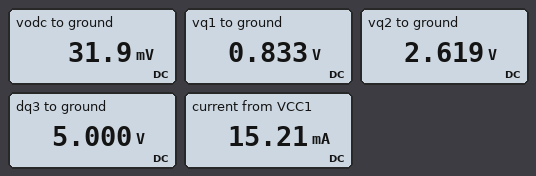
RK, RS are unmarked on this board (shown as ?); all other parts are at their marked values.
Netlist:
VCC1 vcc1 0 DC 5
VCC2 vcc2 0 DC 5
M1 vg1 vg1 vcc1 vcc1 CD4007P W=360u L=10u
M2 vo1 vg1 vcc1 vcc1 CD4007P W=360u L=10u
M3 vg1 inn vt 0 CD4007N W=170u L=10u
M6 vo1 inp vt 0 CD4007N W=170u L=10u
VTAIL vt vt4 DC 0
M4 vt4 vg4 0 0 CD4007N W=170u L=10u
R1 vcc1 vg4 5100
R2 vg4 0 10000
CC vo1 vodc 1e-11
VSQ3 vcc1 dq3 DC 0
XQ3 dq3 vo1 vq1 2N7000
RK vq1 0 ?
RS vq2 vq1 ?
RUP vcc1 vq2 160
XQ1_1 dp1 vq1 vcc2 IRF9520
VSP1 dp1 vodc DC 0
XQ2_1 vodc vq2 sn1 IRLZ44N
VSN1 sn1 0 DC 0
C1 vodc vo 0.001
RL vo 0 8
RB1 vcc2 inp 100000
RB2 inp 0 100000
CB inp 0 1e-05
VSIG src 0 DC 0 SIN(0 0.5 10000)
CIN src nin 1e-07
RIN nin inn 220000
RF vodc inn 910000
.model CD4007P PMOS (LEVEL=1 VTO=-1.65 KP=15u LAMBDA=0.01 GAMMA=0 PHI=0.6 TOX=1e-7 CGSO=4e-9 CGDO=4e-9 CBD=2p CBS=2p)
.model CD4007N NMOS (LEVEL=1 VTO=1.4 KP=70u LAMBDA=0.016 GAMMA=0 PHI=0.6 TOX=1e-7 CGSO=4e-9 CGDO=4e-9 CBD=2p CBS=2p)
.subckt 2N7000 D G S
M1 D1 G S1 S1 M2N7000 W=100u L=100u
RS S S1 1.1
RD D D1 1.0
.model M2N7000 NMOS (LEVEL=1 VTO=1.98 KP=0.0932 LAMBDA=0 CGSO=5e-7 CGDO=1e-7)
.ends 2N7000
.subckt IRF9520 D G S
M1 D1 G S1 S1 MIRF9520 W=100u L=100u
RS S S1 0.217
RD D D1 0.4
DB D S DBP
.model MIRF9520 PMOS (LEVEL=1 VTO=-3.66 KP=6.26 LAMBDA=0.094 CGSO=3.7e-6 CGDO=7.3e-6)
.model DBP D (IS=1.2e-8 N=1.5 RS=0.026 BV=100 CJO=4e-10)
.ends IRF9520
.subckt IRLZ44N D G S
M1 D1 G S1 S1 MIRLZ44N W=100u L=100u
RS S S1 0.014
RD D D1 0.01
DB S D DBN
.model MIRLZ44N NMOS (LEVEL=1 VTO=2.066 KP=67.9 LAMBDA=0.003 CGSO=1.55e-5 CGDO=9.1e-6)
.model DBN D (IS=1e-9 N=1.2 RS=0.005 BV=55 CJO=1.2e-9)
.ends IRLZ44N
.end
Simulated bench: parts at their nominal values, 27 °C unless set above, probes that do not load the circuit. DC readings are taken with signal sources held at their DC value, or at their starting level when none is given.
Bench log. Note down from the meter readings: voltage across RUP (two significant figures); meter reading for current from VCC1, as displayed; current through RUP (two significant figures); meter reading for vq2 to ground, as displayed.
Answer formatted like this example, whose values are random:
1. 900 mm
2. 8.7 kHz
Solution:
1. 2.4 V
2. 15.21 mA
3. 15 mA
4. 2.619 V
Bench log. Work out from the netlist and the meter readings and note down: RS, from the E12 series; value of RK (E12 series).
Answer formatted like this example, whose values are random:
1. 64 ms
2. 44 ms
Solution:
1. 120 Ω
2. 56 Ω
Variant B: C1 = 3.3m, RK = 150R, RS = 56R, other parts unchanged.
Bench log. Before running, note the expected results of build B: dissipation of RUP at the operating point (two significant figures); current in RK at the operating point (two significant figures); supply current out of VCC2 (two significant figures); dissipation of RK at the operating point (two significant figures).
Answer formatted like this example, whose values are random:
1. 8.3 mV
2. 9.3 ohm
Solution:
1. 30 mW
2. 14 mA
3. 25 µA
4. 28 mW
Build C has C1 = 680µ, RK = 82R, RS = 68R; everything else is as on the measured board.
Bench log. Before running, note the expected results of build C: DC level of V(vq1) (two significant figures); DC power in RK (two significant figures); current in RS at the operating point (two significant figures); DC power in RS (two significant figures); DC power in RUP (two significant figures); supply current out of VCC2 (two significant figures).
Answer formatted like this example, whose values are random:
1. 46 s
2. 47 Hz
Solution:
1. 1.3 V
2. 21 mW
3. 16 mA
4. 18 mW
5. 42 mW
6. 1.4 mA
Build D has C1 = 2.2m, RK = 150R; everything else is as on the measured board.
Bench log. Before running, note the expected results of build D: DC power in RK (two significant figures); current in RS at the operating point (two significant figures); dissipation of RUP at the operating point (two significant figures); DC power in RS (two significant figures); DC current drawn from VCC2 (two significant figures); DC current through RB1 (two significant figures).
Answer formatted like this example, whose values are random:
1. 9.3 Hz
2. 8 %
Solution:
1. 20 mW
2. 12 mA
3. 22 mW
4. 16 mW
5. 25 µA
6. 25 µA
